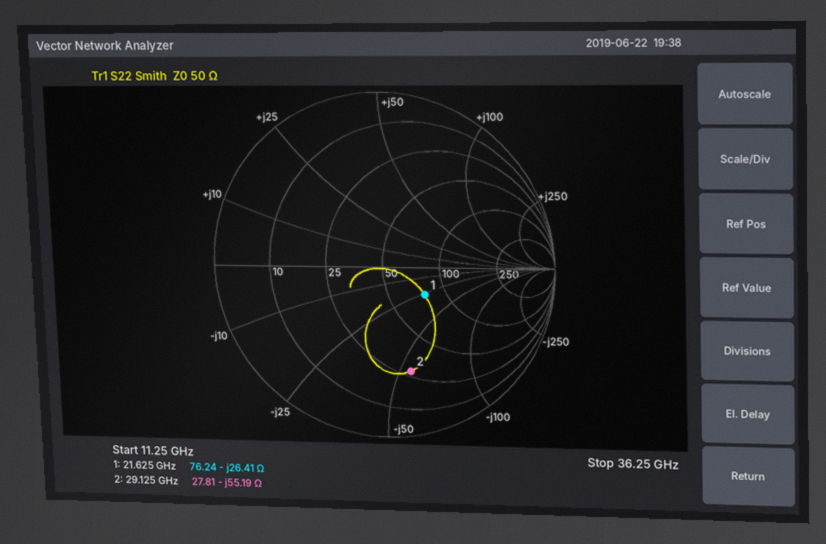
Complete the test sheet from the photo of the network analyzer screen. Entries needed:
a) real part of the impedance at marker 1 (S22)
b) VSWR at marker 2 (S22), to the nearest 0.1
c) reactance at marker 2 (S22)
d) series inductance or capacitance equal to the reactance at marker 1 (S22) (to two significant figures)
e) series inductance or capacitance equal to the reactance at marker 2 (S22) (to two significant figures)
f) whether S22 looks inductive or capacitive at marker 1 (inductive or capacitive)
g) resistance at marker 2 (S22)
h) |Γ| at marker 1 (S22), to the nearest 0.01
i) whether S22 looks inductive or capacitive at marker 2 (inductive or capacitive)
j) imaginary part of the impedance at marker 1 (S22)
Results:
76.24 Ω
4.3
-55.19 Ω
280 fF
99 fF
capacitive
27.81 Ω
0.29
capacitive
-26.41 Ω
